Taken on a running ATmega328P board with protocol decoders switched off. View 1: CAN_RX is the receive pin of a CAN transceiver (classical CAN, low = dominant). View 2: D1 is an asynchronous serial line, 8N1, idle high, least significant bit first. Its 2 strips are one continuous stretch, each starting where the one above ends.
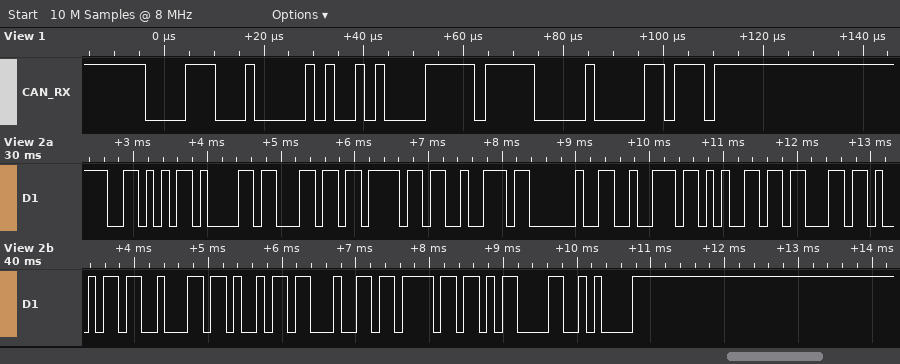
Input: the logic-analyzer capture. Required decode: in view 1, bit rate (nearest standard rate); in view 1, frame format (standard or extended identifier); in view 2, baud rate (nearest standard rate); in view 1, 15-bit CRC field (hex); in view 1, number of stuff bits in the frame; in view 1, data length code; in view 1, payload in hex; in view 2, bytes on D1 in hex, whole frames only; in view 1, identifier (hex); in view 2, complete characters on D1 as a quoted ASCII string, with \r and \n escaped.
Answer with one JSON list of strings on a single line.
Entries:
["500 kbit/s", "standard", "9600 baud", "0x600B", "5", "2", "50 FF", "56 61 6C 6F 72 20 72 65 63 69 62 69 64 6F 0D 0A", "0x0E2", "\"Valor recibido\\r\\n\""]
